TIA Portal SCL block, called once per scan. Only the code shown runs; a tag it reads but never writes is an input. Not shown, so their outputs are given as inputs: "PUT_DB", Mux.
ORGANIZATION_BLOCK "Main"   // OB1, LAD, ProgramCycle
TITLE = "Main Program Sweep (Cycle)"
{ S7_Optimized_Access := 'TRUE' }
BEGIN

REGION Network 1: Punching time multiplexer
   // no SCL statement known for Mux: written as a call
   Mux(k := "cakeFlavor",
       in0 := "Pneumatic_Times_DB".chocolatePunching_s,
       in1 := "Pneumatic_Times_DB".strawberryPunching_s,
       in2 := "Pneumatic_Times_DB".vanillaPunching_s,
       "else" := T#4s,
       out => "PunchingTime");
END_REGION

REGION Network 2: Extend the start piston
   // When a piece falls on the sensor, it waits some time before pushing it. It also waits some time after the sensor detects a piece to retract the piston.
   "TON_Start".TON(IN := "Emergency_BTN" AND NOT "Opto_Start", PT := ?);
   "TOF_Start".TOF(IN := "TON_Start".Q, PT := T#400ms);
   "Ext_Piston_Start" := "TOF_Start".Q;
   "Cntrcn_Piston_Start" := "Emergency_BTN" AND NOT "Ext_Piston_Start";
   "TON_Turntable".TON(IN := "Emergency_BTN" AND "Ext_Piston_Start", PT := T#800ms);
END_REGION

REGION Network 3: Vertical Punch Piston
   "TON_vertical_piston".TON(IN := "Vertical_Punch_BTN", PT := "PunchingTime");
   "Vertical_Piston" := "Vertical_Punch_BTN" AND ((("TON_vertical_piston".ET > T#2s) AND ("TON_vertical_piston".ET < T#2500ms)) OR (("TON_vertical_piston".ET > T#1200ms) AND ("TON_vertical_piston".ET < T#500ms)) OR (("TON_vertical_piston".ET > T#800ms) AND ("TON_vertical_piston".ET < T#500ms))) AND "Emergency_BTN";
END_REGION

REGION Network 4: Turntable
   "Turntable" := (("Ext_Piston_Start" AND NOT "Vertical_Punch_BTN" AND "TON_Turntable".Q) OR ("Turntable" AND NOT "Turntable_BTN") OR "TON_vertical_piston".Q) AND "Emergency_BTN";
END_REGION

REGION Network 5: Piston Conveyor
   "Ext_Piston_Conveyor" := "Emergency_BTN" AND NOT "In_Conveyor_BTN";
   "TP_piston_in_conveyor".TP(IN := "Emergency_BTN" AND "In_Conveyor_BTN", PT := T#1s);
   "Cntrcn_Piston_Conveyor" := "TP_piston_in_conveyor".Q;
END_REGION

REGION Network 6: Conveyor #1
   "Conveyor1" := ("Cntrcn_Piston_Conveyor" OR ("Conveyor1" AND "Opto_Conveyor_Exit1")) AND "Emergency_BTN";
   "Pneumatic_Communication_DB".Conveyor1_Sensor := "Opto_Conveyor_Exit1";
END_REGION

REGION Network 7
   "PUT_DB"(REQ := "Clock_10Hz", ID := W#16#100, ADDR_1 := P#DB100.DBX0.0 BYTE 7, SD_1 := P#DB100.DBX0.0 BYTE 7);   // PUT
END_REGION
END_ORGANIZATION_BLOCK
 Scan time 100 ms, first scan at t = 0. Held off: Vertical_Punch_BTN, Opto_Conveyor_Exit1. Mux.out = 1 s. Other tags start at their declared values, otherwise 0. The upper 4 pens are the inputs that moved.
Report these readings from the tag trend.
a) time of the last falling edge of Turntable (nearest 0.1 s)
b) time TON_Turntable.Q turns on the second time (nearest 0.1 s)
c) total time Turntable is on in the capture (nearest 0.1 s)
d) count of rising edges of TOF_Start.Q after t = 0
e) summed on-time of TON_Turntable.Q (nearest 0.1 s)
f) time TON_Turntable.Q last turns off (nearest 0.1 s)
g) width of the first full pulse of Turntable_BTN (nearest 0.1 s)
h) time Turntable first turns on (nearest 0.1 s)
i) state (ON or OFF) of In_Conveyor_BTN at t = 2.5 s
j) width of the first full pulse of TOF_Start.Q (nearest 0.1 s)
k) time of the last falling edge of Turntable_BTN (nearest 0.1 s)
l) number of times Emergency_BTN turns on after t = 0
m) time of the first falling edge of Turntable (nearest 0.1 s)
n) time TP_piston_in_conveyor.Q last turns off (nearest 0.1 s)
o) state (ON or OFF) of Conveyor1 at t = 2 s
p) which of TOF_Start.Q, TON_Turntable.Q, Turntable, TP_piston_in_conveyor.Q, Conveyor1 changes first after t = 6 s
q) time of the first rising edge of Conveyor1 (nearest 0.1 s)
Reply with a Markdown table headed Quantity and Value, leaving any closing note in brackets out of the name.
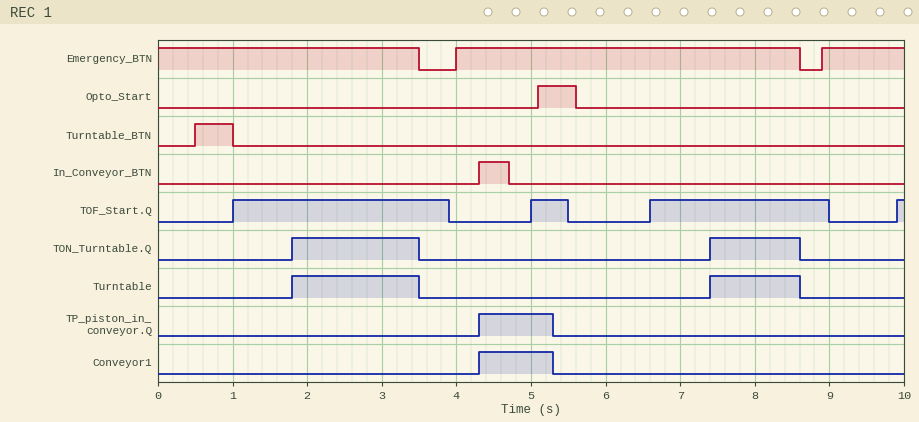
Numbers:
| Quantity | Value |
|---|---|
| time of the last falling edge of Turntable | 8.6 s |
| time TON_Turntable.Q turns on the second time | 7.4 s |
| total time Turntable is on in the capture | 2.9 s |
| count of rising edges of TOF_Start.Q after t = 0 | 4 |
| summed on-time of TON_Turntable.Q | 2.9 s |
| time TON_Turntable.Q last turns off | 8.6 s |
| width of the first full pulse of Turntable_BTN | 0.5 s |
| time Turntable first turns on | 1.8 s |
| state (ON or OFF) of In_Conveyor_BTN at t = 2.5 s | OFF |
| width of the first full pulse of TOF_Start.Q | 2.9 s |
| time of the last falling edge of Turntable_BTN | 1.0 s |
| number of times Emergency_BTN turns on after t = 0 | 2 |
| time of the first falling edge of Turntable | 3.5 s |
| time TP_piston_in_conveyor.Q last turns off | 5.3 s |
| state (ON or OFF) of Conveyor1 at t = 2 s | OFF |
| which of TOF_Start.Q, TON_Turntable.Q, Turntable, TP_piston_in_conveyor.Q, Conveyor1 changes first after t = 6 s | TOF_Start.Q |
| time of the first rising edge of Conveyor1 | 4.3 s |
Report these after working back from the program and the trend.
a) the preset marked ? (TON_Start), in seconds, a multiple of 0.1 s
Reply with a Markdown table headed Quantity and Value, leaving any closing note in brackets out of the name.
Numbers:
| Quantity | Value |
|---|---|
| the preset marked ? (TON_Start), in seconds, a multiple of 0.1 s | 1.0 s |
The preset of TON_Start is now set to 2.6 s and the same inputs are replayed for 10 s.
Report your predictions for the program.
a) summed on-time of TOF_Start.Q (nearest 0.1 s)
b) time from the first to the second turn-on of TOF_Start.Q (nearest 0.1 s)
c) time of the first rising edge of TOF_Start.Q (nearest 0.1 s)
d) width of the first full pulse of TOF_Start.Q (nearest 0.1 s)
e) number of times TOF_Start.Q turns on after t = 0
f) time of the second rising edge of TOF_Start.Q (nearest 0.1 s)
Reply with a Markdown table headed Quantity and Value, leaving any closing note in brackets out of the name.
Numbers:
| Quantity | Value |
|---|---|
| summed on-time of TOF_Start.Q | 2.1 s |
| time from the first to the second turn-on of TOF_Start.Q | 5.6 s |
| time of the first rising edge of TOF_Start.Q | 2.6 s |
| width of the first full pulse of TOF_Start.Q | 1.3 s |
| number of times TOF_Start.Q turns on after t = 0 | 2 |
| time of the second rising edge of TOF_Start.Q | 8.2 s |
